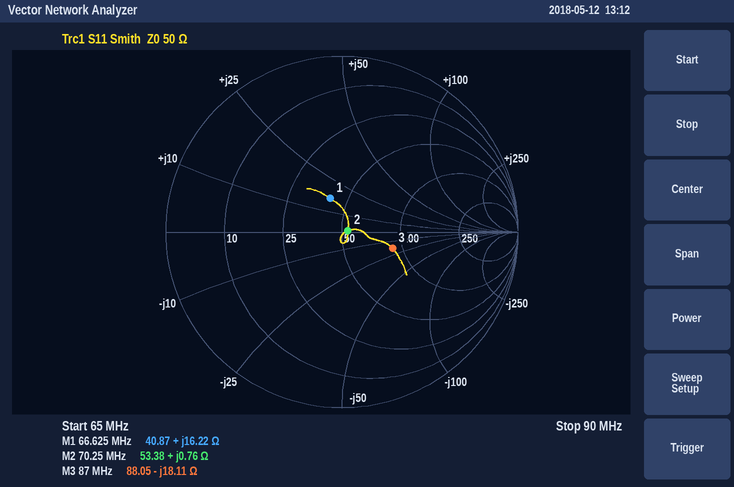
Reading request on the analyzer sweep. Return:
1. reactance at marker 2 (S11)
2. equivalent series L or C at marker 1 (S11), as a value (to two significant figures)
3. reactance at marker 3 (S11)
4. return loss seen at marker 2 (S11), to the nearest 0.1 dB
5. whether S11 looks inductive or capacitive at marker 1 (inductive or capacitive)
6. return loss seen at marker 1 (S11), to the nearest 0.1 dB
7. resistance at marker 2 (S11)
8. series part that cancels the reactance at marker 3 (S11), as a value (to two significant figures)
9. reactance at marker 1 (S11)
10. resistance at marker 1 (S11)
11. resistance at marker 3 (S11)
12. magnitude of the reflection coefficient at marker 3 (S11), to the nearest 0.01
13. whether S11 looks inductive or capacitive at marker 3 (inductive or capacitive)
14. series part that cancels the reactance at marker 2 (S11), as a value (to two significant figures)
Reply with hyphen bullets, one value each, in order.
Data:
- +0.76 Ω
- 39 nH
- -18.11 Ω
- 29.5 dB
- inductive
- 13.9 dB
- 53.38 Ω
- 33 nH
- +16.22 Ω
- 40.87 Ω
- 88.05 Ω
- 0.30
- capacitive
- 3.0 nF
